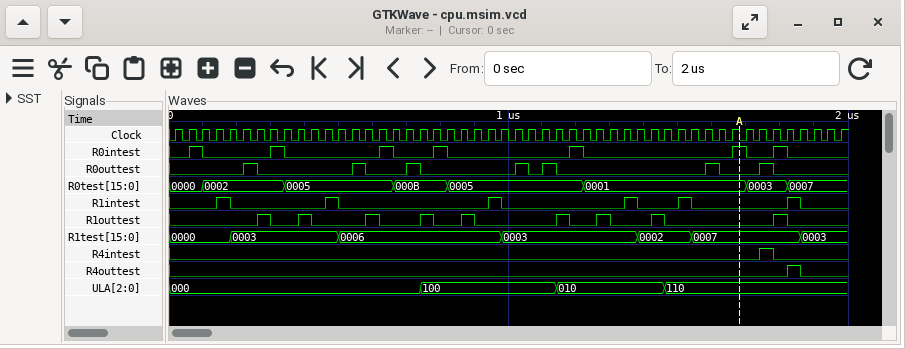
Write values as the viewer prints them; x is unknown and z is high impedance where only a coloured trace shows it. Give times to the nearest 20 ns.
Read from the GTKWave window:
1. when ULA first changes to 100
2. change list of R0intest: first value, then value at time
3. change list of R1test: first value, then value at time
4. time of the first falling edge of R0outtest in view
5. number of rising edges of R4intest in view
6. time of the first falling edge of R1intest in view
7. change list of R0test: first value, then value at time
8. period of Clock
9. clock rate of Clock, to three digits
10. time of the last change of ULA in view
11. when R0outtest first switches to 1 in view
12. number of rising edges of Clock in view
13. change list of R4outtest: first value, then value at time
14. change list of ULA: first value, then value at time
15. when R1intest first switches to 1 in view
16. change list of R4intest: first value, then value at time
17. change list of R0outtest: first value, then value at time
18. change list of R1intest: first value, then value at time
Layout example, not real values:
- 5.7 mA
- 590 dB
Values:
- 740 ns
- 0, 1 at 60 ns, 0 at 100 ns, 1 at 300 ns, 0 at 340 ns, 1 at 620 ns, 0 at 660 ns, 1 at 780 ns, 0 at 820 ns, 1 at 1180 ns, 0 at 1220 ns, 1 at 1660 ns, 0 at 1700 ns, 1 at 1780 ns, 0 at 1820 ns
- 0000, 0003 at 180 ns, 0006 at 500 ns, 0003 at 980 ns, 0002 at 1380 ns, 0007 at 1540 ns, 0003 at 1860 ns
- 260 ns
- 1
- 180 ns
- 0000, 0002 at 100 ns, 0005 at 340 ns, 000B at 660 ns, 0005 at 820 ns, 0001 at 1220 ns, 0003 at 1700 ns, 0007 at 1820 ns
- 40 ns
- 25.0 MHz
- 1460 ns
- 220 ns
- 50
- 0, 1 at 1820 ns, 0 at 1860 ns
- 000, 100 at 740 ns, 010 at 1140 ns, 110 at 1460 ns
- 140 ns
- 0, 1 at 1740 ns, 0 at 1780 ns
- 0, 1 at 220 ns, 0 at 260 ns, 1 at 540 ns, 0 at 580 ns, 1 at 700 ns, 0 at 740 ns, 1 at 1020 ns, 0 at 1060 ns, 1 at 1100 ns, 0 at 1140 ns, 1 at 1580 ns, 0 at 1620 ns, 1 at 1740 ns, 0 at 1780 ns
- 0, 1 at 140 ns, 0 at 180 ns, 1 at 460 ns, 0 at 500 ns, 1 at 940 ns, 0 at 980 ns, 1 at 1340 ns, 0 at 1380 ns, 1 at 1500 ns, 0 at 1540 ns, 1 at 1820 ns, 0 at 1860 ns
